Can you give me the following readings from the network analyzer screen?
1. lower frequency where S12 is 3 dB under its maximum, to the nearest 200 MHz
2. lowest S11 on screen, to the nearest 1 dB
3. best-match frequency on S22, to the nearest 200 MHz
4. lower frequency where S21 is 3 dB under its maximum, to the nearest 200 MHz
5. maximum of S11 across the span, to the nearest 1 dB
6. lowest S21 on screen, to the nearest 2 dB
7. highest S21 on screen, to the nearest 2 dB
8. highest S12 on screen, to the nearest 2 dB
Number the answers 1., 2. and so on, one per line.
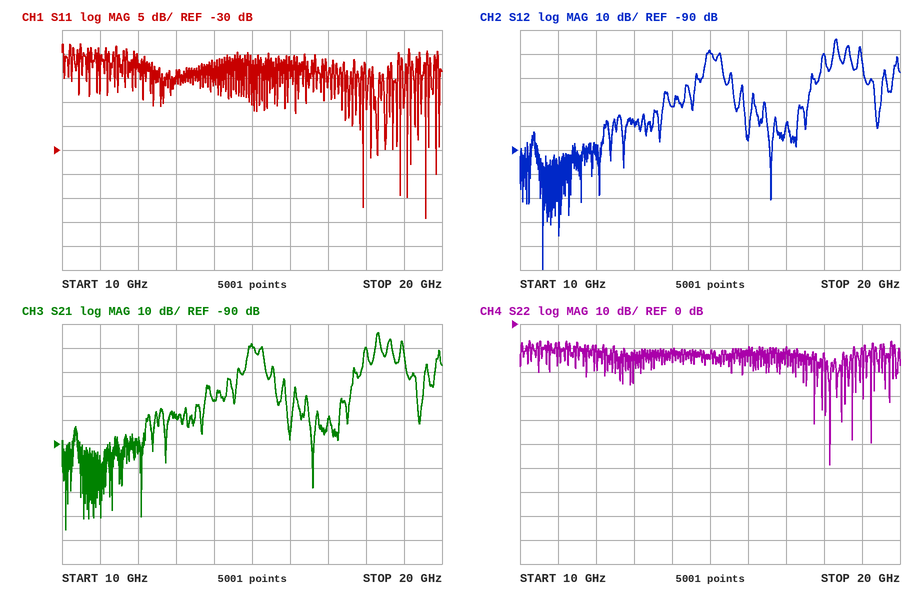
1. 18.2 GHz
2. -44 dB
3. 18.2 GHz
4. 18.2 GHz
5. -8 dB
6. -126 dB
7. -44 dB
8. -44 dB
